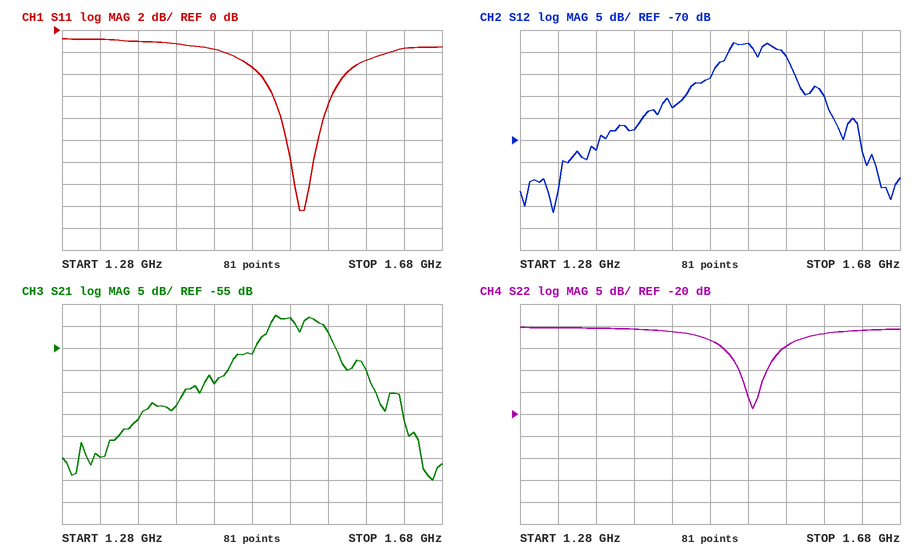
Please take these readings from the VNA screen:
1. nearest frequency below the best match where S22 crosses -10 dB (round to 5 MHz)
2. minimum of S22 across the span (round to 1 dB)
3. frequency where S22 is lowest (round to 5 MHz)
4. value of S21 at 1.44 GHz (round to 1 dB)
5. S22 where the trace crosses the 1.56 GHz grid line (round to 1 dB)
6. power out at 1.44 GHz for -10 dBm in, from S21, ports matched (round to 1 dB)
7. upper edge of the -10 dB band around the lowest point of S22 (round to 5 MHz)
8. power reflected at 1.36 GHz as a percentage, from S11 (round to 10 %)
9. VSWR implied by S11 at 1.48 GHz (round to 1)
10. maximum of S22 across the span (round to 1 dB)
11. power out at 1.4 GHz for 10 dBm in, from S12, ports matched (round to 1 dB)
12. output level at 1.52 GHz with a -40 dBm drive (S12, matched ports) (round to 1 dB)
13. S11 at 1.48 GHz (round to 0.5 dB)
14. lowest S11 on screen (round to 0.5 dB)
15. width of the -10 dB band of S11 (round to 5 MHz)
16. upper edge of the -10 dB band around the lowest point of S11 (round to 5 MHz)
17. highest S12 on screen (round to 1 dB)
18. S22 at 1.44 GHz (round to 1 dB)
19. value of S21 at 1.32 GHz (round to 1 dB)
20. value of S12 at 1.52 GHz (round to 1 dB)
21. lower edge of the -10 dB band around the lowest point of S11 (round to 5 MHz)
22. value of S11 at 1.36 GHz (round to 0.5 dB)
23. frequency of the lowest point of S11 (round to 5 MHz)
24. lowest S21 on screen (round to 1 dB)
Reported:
1.510 GHz
-19 dB
1.525 GHz
-63 dB
-5 dB
-73 dBm
1.540 GHz
80 %
5
0 dB
-58 dBm
-88 dBm
-3.5 dB
-16.5 dB
35 MHz
1.550 GHz
-48 dB
-1 dB
-80 dB
-48 dB
1.515 GHz
-1.0 dB
1.530 GHz
-85 dB
